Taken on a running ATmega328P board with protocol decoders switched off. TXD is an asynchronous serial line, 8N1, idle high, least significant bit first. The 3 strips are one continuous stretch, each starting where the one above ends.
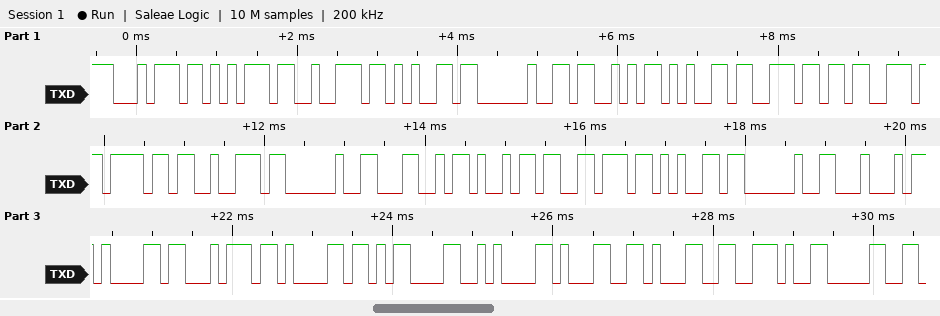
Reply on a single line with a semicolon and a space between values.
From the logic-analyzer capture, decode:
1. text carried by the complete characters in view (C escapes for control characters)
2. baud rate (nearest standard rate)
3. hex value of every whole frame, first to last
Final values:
"ture Sensor Live Data\r\n11.0"; 9600 baud; 0x74 0x75 0x72 0x65 0x20 0x53 0x65 0x6E 0x73 0x6F 0x72 0x20 0x4C 0x69 0x76 0x65 0x20 0x44 0x61 0x74 0x61 0x0D 0x0A 0x31 0x31 0x2E 0x30
